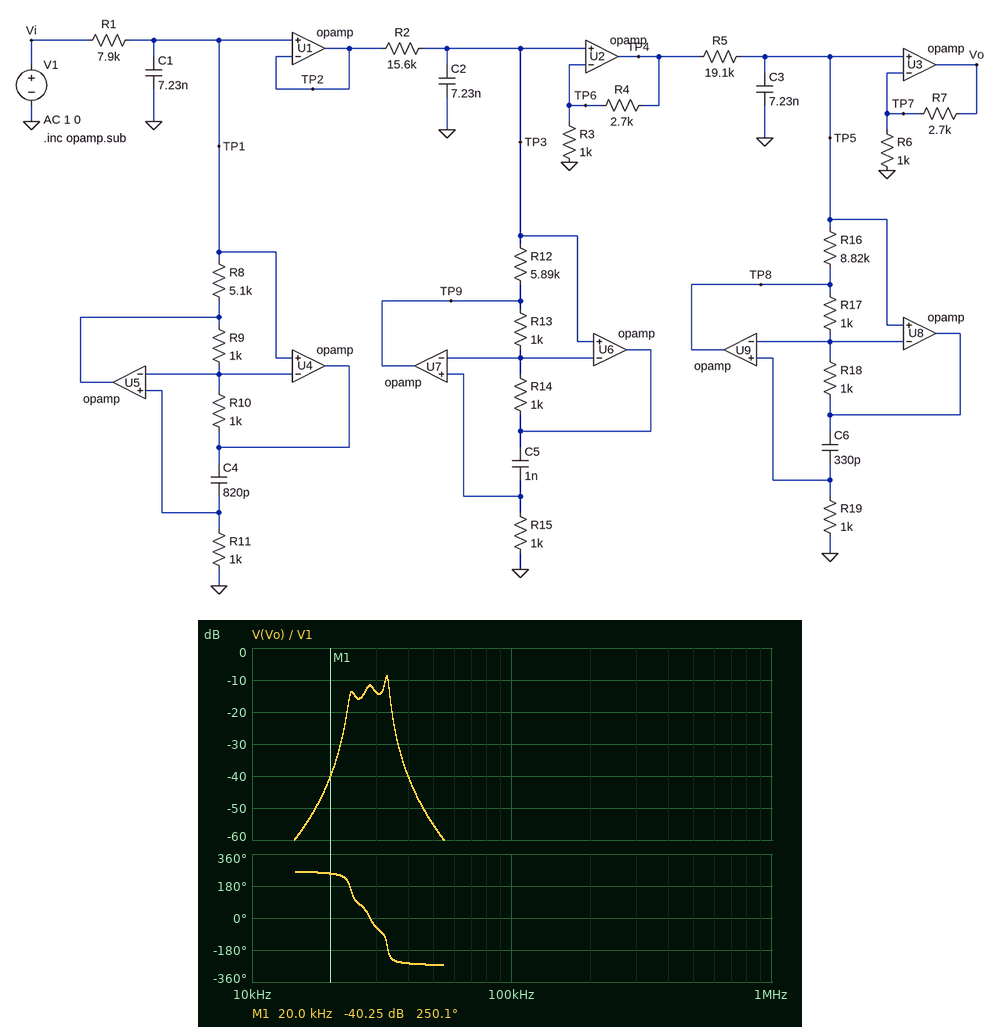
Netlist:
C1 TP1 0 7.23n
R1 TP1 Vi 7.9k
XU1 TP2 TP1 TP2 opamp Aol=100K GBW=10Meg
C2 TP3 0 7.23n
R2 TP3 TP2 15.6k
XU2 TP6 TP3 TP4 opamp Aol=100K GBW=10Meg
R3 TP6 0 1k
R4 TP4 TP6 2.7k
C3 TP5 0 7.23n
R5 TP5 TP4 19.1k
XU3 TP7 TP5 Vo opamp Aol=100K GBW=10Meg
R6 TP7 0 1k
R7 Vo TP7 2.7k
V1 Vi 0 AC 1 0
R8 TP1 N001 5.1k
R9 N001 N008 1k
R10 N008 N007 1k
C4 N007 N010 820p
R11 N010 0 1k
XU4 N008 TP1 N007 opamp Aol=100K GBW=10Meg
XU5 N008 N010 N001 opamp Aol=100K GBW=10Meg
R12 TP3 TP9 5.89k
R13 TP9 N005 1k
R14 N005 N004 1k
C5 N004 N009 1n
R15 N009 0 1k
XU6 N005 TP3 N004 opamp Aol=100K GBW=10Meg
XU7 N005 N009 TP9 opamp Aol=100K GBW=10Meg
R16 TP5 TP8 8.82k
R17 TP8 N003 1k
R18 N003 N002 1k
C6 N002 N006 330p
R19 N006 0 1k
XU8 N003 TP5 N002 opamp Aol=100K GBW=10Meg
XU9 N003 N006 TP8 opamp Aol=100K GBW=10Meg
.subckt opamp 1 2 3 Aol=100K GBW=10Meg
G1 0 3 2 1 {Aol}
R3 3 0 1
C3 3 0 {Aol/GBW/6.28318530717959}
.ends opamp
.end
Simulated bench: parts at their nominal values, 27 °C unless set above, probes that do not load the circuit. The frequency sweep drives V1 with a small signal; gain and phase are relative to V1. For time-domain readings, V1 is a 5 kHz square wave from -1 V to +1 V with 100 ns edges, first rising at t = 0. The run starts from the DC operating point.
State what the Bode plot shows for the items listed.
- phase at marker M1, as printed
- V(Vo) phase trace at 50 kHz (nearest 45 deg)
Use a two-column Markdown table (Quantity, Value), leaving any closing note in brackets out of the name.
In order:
| Quantity | Value |
|---|---|
| phase at marker M1, as printed | 250.1 deg |
| V(Vo) phase trace at 50 kHz | -270 deg |
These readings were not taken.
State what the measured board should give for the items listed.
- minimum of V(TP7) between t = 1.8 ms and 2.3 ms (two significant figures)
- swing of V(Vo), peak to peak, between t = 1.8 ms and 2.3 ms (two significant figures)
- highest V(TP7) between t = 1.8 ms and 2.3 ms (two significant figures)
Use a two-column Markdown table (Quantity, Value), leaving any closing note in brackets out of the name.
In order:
| Quantity | Value |
|---|---|
| minimum of V(TP7) between t = 1.8 ms and 2.3 ms | -15 mV |
| swing of V(Vo), peak to peak, between t = 1.8 ms and 2.3 ms | 110 mV |
| highest V(TP7) between t = 1.8 ms and 2.3 ms | 15 mV |
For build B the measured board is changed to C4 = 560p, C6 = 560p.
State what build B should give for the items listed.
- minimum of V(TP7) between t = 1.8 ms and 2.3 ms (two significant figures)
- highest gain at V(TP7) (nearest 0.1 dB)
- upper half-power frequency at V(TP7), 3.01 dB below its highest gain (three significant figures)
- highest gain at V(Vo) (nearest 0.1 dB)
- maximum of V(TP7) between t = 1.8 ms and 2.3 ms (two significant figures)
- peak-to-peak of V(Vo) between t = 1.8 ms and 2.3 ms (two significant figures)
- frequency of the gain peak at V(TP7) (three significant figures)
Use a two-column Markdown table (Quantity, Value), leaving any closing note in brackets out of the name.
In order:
| Quantity | Value |
|---|---|
| minimum of V(TP7) between t = 1.8 ms and 2.3 ms | -41 mV |
| highest gain at V(TP7) | -14.2 dB |
| upper half-power frequency at V(TP7), 3.01 dB below its highest gain | 26.3 kHz |
| highest gain at V(Vo) | -2.8 dB |
| maximum of V(TP7) between t = 1.8 ms and 2.3 ms | 41 mV |
| peak-to-peak of V(Vo) between t = 1.8 ms and 2.3 ms | 300 mV |
| frequency of the gain peak at V(TP7) | 25.8 kHz |
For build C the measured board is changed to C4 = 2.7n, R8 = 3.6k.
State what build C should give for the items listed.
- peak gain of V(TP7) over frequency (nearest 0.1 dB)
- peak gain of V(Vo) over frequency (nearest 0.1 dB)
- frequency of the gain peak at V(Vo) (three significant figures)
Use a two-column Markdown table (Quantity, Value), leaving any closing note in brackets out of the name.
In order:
| Quantity | Value |
|---|---|
| peak gain of V(TP7) over frequency | -24.9 dB |
| peak gain of V(Vo) over frequency | -13.6 dB |
| frequency of the gain peak at V(Vo) | 24.0 kHz |
